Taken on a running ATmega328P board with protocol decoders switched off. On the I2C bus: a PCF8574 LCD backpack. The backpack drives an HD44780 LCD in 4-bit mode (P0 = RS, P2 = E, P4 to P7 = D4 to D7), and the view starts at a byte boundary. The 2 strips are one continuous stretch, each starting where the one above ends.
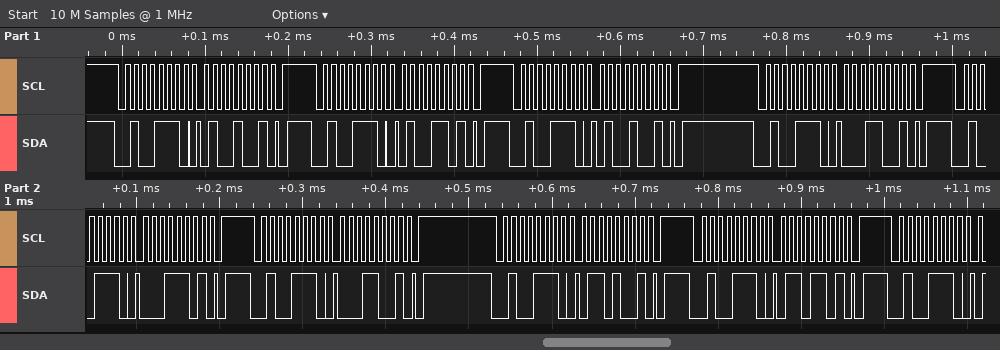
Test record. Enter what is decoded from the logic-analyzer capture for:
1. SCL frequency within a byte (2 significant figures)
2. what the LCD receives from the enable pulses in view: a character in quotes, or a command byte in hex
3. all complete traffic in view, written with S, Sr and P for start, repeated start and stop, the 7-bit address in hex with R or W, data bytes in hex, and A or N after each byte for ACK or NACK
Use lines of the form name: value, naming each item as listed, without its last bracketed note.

SCL frequency within a byte: 100 kHz
what the LCD receives from the enable pulses in view: a character in quotes, or a command byte in hex: 'A'
all complete traffic in view, written with S, Sr and P for start, repeated start and stop, the 7-bit address in hex with R or W, data bytes in hex, and A or N after each byte for ACK or NACK: S 27W A 49 A P S 27W A 4D A P S 27W A 49 A P S 27W A 19 A P S 27W A 1D A P S 27W A 19 A P S 27W A 69 A P S 27W A 6D A P S 27W A
